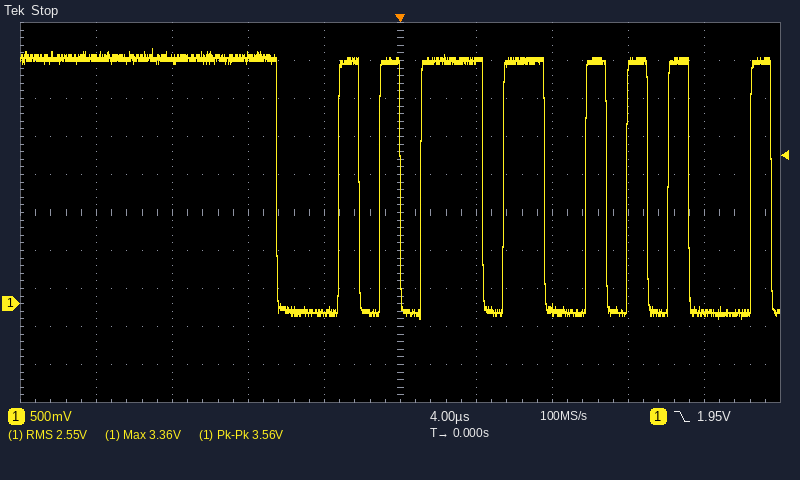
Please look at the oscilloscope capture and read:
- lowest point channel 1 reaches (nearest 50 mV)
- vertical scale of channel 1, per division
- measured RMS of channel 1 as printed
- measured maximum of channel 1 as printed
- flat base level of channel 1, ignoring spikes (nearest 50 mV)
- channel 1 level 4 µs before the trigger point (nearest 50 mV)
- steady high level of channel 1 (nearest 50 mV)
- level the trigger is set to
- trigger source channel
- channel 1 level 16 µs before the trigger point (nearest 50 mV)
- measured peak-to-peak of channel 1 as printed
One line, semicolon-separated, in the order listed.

-200 mV; 500 mV; 2.55 V; 3.36 V; -100 mV; -100 mV; 3.20 V; 1.95 V; channel 1; 3.25 V; 3.56 V
